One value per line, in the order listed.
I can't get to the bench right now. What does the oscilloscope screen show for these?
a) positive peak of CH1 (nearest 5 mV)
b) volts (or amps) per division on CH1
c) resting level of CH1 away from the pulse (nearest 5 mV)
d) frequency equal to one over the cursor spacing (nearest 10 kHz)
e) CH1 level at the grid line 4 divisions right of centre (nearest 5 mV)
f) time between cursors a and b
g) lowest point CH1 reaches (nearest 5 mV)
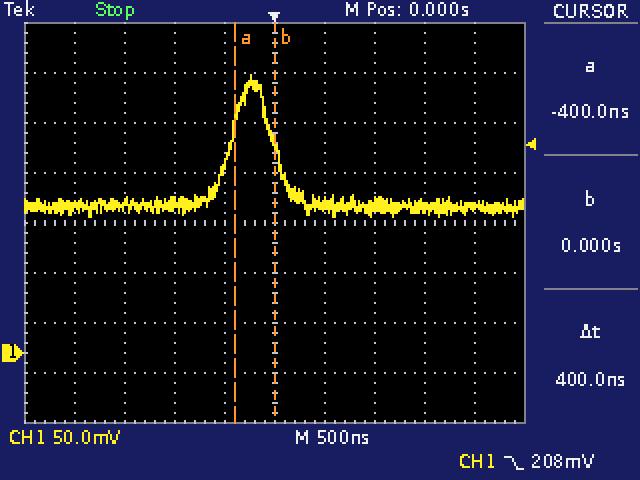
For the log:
280 mV
50 mV
145 mV
2.50 MHz
145 mV
400 ns
135 mV
